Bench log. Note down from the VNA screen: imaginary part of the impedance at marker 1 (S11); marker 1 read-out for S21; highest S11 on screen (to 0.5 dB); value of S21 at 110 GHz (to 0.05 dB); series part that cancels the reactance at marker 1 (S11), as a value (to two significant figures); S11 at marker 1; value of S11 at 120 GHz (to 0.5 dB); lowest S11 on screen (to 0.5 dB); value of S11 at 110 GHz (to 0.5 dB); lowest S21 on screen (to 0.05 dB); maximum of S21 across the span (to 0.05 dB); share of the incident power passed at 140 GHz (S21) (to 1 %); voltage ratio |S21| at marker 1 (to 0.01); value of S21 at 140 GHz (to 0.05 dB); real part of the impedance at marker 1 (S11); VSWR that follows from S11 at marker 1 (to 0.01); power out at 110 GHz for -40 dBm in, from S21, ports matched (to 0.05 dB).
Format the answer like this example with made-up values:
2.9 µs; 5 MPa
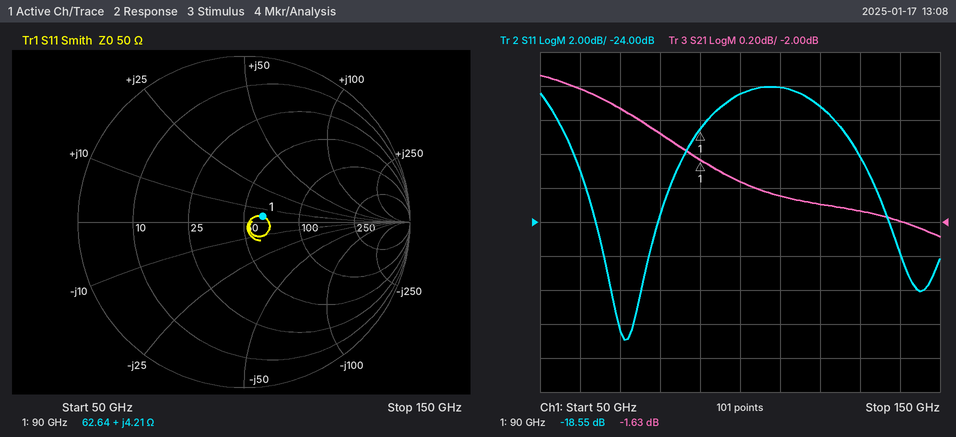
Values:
+4.21 Ω; -1.63 dB; -16.0 dB; -1.85 dB; 420 fF; -18.55 dB; -17.0 dB; -31.0 dB; -16.0 dB; -2.10 dB; -1.15 dB; 63 %; 0.83; -2.00 dB; 62.64 Ω; 1.27; -41.85 dBm
